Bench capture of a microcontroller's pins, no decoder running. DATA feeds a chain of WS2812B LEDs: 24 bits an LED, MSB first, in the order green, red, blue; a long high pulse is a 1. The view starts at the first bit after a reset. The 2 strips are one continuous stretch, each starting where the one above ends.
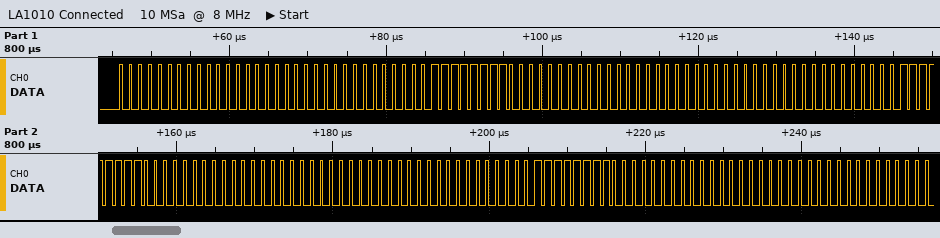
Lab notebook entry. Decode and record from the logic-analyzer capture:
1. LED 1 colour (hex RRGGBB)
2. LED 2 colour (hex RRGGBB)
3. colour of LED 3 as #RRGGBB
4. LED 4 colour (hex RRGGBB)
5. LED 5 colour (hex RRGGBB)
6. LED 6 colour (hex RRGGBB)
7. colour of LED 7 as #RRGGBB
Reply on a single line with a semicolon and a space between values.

#000000; #FF0000; #000000; #FF0000; #000000; #FF0000; #000000
